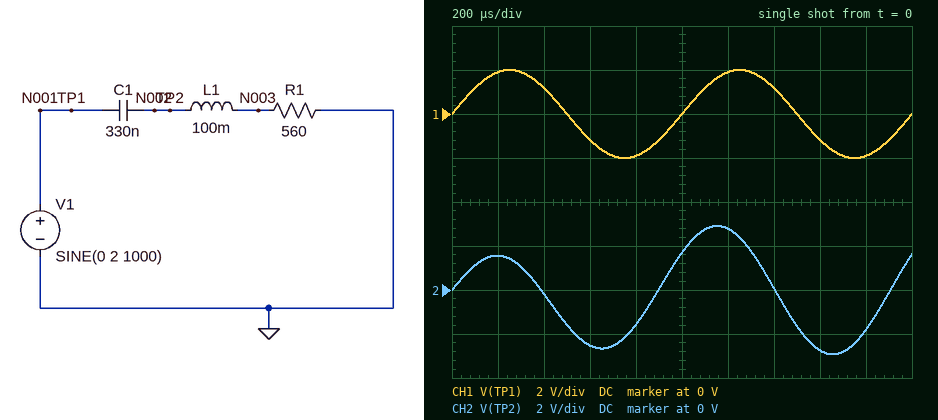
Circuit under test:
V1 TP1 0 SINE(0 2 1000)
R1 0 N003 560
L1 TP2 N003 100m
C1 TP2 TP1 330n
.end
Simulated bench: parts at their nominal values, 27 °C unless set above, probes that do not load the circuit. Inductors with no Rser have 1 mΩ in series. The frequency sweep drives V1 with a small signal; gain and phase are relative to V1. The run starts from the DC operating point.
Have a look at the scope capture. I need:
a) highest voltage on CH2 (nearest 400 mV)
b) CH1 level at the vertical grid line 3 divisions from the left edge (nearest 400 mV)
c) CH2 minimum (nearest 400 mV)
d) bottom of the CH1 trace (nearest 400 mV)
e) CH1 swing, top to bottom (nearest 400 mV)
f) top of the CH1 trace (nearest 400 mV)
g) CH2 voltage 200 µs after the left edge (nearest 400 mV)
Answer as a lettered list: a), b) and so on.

a) 2.8 V
b) -1.2 V
c) -2.8 V
d) -2.0 V
e) 4.0 V
f) 2.0 V
g) 1.6 V
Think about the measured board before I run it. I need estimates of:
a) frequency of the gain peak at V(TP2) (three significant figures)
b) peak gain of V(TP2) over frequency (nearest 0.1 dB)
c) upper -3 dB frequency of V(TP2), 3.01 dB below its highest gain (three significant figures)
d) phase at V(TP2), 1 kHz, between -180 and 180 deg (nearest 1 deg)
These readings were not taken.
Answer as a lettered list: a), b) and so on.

a) 1.03 kHz
b) 3.3 dB
c) 5.11 kHz
d) 34 deg
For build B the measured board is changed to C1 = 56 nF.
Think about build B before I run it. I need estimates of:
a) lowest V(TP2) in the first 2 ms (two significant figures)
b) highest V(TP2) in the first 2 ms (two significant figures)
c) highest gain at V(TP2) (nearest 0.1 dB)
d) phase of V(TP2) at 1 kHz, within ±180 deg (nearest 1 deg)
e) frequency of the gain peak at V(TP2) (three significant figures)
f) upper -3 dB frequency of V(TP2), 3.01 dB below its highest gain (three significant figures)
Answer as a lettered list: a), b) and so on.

a) -1.1 V
b) 900 mV
c) 8.4 dB
d) 124 deg
e) 2.21 kHz
f) 2.93 kHz
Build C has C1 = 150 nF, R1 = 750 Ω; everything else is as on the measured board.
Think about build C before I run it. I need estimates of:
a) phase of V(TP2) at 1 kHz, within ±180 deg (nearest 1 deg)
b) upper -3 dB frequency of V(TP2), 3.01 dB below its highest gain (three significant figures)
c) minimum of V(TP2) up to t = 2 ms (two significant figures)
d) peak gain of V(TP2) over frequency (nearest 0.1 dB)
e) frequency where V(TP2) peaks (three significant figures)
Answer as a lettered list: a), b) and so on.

a) 70 deg
b) 4.52 kHz
c) -2.3 V
d) 3.7 dB
e) 1.49 kHz
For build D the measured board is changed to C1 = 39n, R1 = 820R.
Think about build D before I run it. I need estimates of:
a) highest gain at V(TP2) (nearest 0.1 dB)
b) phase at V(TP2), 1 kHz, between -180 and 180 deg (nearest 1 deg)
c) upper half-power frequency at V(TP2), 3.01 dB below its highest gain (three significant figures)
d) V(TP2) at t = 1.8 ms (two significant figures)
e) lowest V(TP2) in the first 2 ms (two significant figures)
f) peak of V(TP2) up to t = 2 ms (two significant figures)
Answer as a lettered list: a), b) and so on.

a) 7.0 dB
b) 114 deg
c) 3.91 kHz
d) 390 mV
e) -730 mV
f) 790 mV
